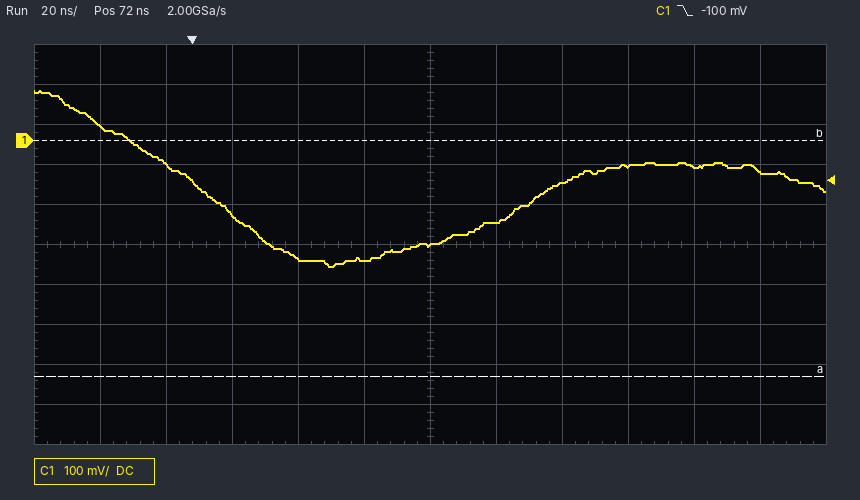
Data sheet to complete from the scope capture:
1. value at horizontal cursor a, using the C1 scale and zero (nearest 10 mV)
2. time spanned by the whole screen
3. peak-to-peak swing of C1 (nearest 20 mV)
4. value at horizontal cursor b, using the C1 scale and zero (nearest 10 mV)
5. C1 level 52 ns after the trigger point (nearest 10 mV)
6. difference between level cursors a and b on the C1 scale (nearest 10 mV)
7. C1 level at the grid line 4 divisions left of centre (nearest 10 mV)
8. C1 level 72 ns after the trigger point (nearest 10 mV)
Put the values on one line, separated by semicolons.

-590 mV; 240 ns; 440 mV; 0 mV; -300 mV; 590 mV; -60 mV; -260 mV
